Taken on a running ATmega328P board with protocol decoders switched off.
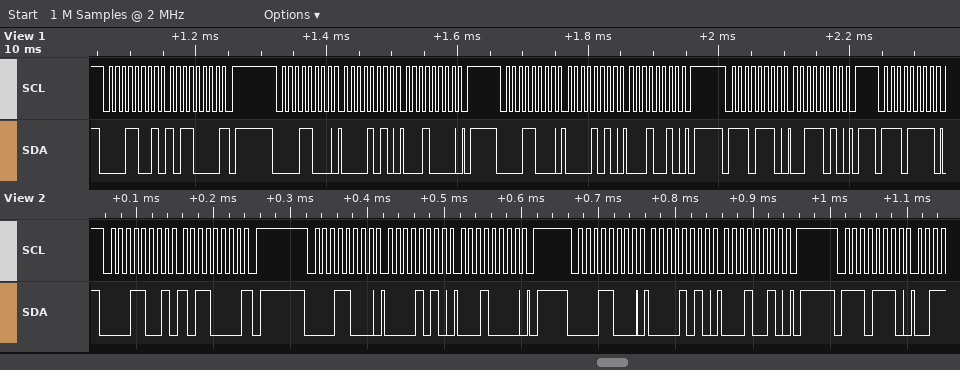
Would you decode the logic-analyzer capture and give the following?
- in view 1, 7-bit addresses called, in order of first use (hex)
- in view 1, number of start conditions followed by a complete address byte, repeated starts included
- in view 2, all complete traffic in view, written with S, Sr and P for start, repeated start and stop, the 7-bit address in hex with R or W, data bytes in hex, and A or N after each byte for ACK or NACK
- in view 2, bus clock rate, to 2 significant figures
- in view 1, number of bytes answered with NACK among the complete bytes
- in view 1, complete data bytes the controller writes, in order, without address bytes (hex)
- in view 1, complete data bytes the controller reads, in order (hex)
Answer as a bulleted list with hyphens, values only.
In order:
- 0x0C 0x77
- 5
- S 0CR A B0 N P S 0CW A 0A A 10 A P S 0CW A 0A A 12 A P S 77W A
- 100 kHz
- 1
- 0A 10 0A 12 3A
- B0
